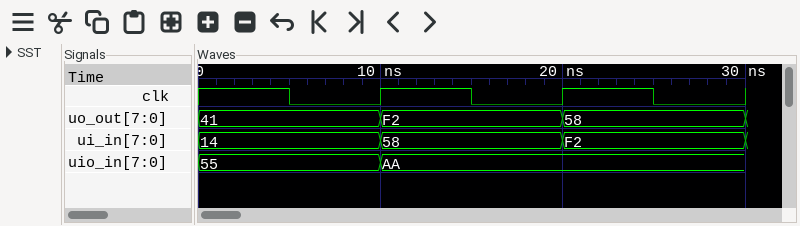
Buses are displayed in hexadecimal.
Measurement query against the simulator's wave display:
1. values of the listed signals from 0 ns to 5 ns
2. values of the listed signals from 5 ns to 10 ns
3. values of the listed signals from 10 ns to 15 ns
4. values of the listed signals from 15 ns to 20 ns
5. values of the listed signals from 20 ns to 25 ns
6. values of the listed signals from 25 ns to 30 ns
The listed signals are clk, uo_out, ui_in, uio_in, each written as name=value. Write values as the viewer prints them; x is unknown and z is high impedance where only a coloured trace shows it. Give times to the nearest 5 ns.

clk=1, uo_out=41, ui_in=14, uio_in=55
clk=0, uo_out=41, ui_in=14, uio_in=55
clk=1, uo_out=F2, ui_in=58, uio_in=AA
clk=0, uo_out=F2, ui_in=58, uio_in=AA
clk=1, uo_out=58, ui_in=F2, uio_in=AA
clk=0, uo_out=58, ui_in=F2, uio_in=AA
